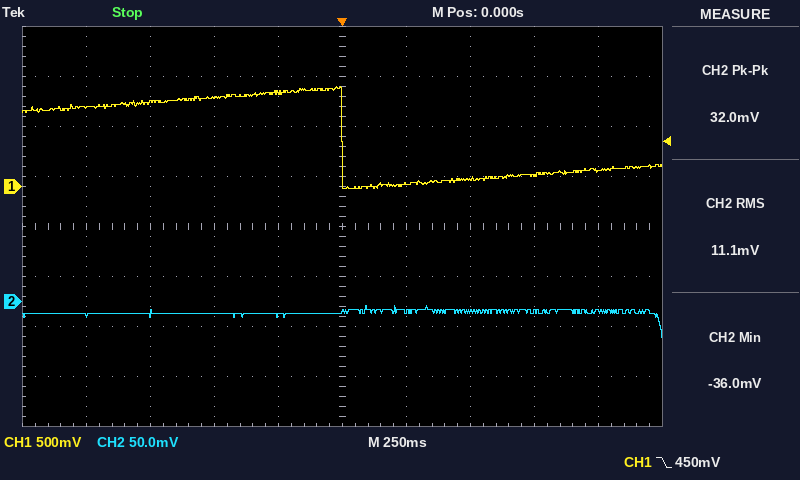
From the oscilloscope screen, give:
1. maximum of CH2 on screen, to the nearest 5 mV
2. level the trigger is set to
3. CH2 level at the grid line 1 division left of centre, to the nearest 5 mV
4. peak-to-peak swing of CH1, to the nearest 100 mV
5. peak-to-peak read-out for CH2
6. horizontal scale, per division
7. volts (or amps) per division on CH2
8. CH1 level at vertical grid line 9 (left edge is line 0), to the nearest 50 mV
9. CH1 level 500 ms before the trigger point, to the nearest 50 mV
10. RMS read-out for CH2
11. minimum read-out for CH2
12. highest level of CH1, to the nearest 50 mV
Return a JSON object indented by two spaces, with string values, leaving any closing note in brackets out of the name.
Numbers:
{
  "maximum of CH2 on screen, to the nearest 5 mV": "-5 mV",
  "level the trigger is set to": "450 mV",
  "CH2 level at the grid line 1 division left of centre, to the nearest 5 mV": "-15 mV",
  "peak-to-peak swing of CH1, to the nearest 100 mV": "1.00 V",
  "peak-to-peak read-out for CH2": "32.0 mV",
  "horizontal scale, per division": "250 ms",
  "volts (or amps) per division on CH2": "50 mV",
  "CH1 level at vertical grid line 9 (left edge is line 0), to the nearest 50 mV": "150 mV",
  "CH1 level 500 ms before the trigger point, to the nearest 50 mV": "900 mV",
  "RMS read-out for CH2": "11.1 mV",
  "minimum read-out for CH2": "-36.0 mV",
  "highest level of CH1, to the nearest 50 mV": "1.00 V"
}
